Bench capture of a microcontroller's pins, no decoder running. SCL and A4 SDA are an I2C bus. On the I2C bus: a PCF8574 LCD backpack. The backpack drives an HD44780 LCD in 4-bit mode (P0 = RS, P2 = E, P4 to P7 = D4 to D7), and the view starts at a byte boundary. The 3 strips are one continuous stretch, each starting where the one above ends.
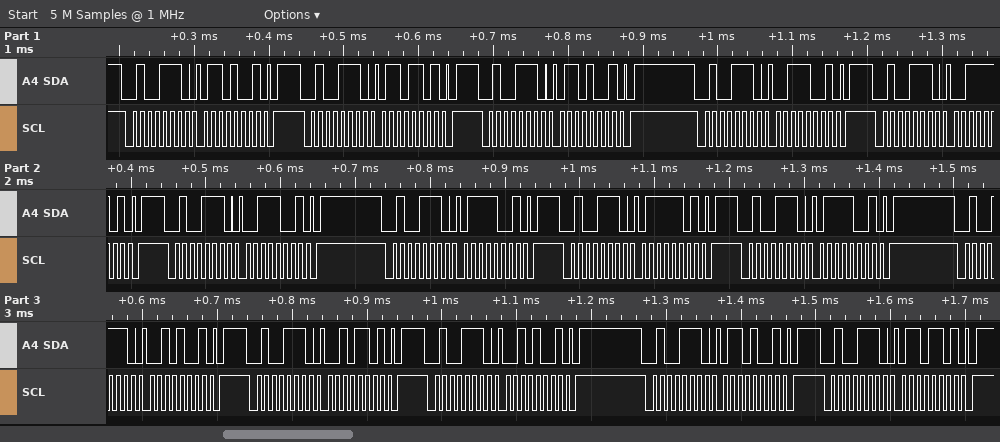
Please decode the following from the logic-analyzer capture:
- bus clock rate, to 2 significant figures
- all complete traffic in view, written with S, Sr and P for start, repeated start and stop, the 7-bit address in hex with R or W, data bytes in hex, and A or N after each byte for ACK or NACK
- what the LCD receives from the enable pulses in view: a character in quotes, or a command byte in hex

100 kHz
S 27W A 69 A P S 27W A 6D A P S 27W A 69 A P S 27W A 39 A P S 27W A 3D A P S 27W A 39 A P S 27W A 79 A P S 27W A 7D A P S 27W A 79 A P S 27W A 29 A P S 27W A 2D A P S 27W A 29 A P S 27W A 69 A P S 27W A 6D A P
'c' 'r'
